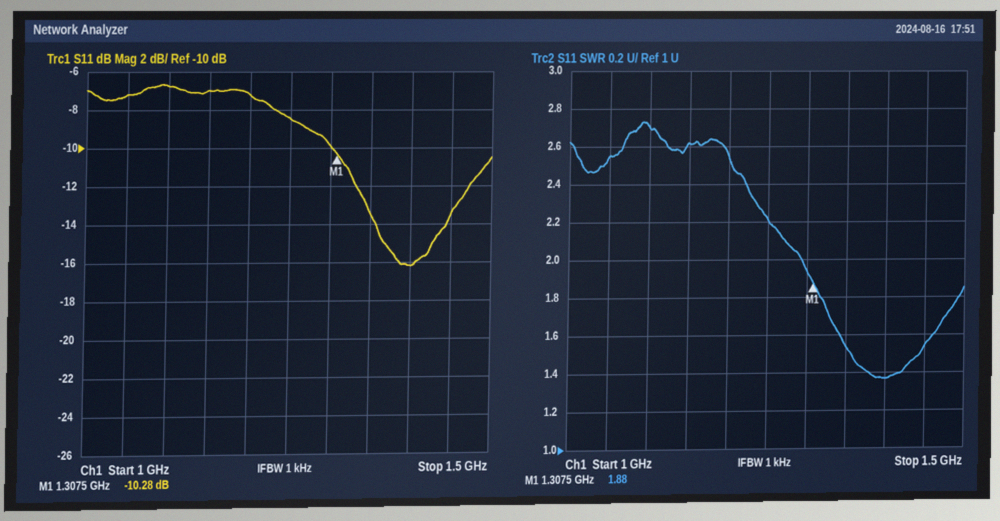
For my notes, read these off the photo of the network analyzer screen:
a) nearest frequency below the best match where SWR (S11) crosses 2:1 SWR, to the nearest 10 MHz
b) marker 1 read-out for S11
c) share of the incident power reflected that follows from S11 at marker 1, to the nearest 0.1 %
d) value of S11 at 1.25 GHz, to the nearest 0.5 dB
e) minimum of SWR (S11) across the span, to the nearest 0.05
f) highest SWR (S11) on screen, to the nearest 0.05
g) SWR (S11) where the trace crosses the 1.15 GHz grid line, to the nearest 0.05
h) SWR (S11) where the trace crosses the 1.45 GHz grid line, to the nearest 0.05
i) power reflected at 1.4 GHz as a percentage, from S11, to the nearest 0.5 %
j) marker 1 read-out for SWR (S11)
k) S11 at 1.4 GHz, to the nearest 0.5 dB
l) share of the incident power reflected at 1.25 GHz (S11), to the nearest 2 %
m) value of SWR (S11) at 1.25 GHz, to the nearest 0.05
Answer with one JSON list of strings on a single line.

["1.29 GHz", "-10.28 dB", "9.4 %", "-8.5 dB", "1.35", "2.75", "2.60", "1.55", "2.5 %", "1.88", "-16.0 dB", "14 %", "2.20"]
